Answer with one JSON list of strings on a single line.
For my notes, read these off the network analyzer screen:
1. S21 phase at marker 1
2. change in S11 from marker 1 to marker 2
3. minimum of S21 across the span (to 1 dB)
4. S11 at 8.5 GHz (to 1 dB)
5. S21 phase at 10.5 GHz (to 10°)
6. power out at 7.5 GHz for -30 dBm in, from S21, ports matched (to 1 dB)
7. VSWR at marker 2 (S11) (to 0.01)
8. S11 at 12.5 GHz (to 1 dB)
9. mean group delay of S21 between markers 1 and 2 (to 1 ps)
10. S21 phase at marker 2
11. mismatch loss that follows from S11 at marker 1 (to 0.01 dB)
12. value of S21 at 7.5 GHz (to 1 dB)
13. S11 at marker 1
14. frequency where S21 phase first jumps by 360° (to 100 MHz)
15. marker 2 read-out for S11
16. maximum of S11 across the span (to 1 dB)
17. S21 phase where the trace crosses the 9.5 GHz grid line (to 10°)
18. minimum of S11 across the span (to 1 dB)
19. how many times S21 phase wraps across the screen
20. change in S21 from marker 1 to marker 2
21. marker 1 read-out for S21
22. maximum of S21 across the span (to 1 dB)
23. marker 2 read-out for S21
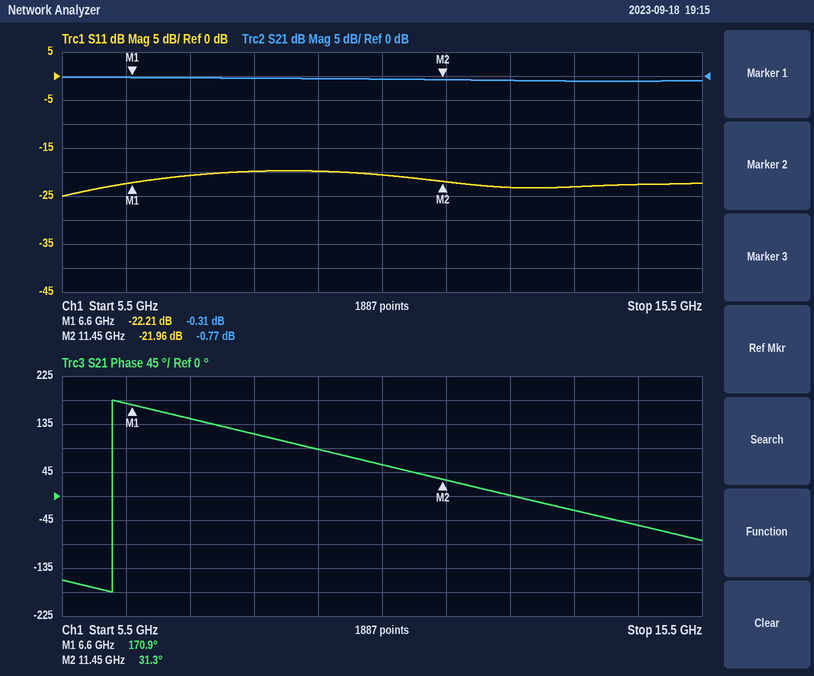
["170.9°", "0.25 dB", "-1 dB", "-20 dB", "60°", "-30 dBm", "1.17", "-23 dB", "80 ps", "31.3°", "0.03 dB", "0 dB", "-22.21 dB", "6.3 GHz", "-21.96 dB", "-20 dB", "90°", "-25 dB", "1", "-0.46 dB", "-0.31 dB", "0 dB", "-0.77 dB"]
